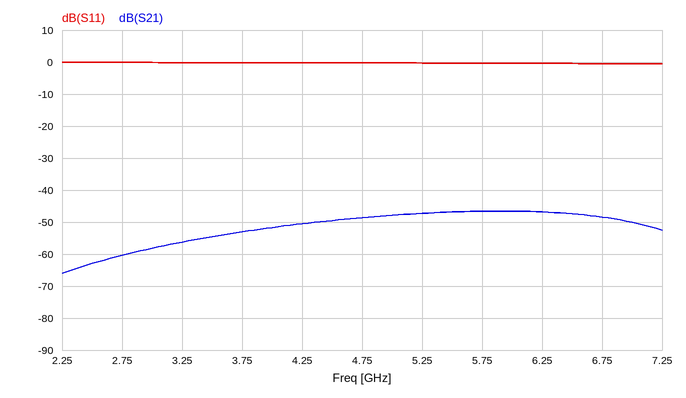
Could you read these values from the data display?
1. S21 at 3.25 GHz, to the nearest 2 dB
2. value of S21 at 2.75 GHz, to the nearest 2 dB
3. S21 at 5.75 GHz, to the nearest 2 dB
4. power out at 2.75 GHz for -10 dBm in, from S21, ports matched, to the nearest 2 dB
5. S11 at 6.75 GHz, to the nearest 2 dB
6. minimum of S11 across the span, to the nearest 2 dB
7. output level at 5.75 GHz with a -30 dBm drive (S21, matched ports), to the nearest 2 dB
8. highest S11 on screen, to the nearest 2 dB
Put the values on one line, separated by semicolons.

-56 dB; -60 dB; -46 dB; -70 dBm; 0 dB; 0 dB; -76 dBm; 0 dB
